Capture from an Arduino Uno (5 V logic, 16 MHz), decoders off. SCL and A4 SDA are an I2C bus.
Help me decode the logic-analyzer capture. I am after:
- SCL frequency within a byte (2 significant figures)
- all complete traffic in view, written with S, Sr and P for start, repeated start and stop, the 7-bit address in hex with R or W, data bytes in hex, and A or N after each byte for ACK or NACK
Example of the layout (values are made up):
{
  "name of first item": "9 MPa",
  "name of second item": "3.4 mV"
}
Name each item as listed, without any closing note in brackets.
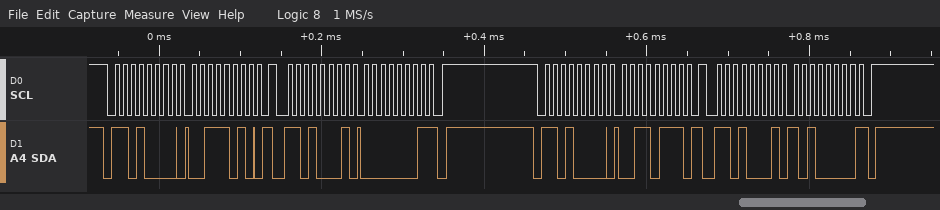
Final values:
{
  "SCL frequency within a byte": "100 kHz",
  "all complete traffic in view, written with S, Sr and P for start, repeated start and stop, the 7-bit address in hex with R or W, data bytes in hex, and A or N after each byte for ACK or NACK": "S 68W A 3A A Sr 68R A 01 N P S 68W A 37 A Sr 68R A A0 N P"
}
